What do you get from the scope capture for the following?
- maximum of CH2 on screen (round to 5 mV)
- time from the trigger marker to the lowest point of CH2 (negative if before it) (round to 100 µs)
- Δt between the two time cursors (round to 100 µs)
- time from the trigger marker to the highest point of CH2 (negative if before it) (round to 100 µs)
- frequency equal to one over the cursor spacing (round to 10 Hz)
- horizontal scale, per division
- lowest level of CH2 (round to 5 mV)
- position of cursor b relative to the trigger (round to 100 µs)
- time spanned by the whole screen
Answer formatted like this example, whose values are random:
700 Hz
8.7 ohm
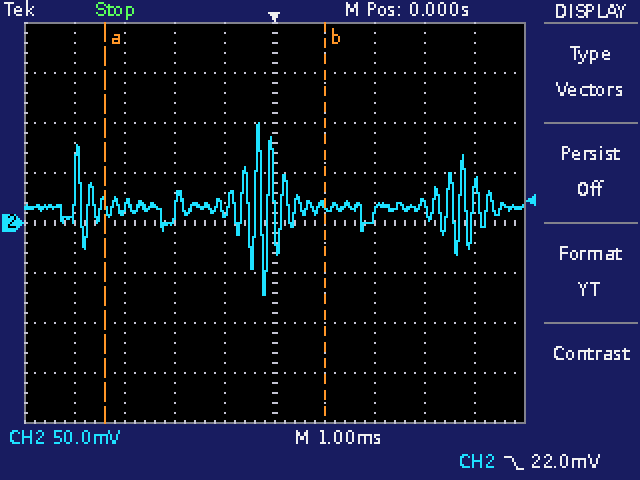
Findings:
100 mV
-200 µs
4.4 ms
-300 µs
230 Hz
1 ms
-70 mV
+1.0 ms
10 ms
